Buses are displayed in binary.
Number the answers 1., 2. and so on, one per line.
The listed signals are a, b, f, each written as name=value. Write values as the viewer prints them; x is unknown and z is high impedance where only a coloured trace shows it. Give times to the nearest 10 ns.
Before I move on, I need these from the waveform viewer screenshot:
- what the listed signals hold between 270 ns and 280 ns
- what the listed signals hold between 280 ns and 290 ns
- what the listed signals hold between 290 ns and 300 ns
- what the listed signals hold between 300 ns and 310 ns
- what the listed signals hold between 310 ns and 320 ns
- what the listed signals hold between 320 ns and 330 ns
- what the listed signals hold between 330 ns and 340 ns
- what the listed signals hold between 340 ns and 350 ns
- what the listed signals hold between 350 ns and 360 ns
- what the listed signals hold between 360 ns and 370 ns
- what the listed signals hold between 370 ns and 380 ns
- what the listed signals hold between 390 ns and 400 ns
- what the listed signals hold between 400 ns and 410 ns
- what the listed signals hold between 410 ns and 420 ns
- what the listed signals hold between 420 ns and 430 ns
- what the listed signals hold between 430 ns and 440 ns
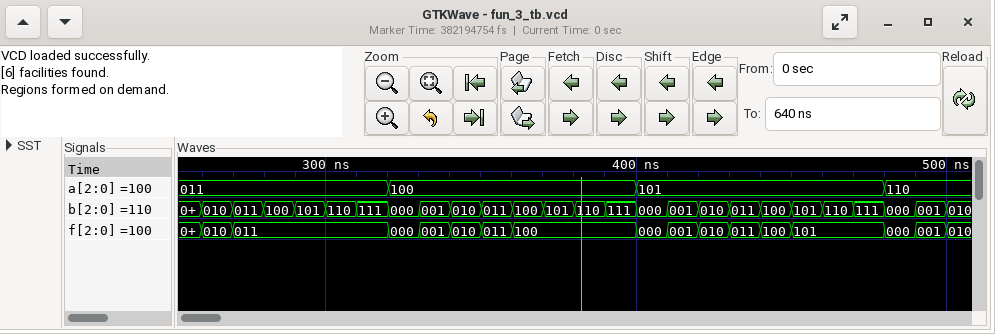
1. a=011, b=011, f=011
2. a=011, b=100, f=011
3. a=011, b=101, f=011
4. a=011, b=110, f=011
5. a=011, b=111, f=011
6. a=100, b=000, f=000
7. a=100, b=001, f=001
8. a=100, b=010, f=010
9. a=100, b=011, f=011
10. a=100, b=100, f=100
11. a=100, b=101, f=100
12. a=100, b=111, f=100
13. a=101, b=000, f=000
14. a=101, b=001, f=001
15. a=101, b=010, f=010
16. a=101, b=011, f=011
